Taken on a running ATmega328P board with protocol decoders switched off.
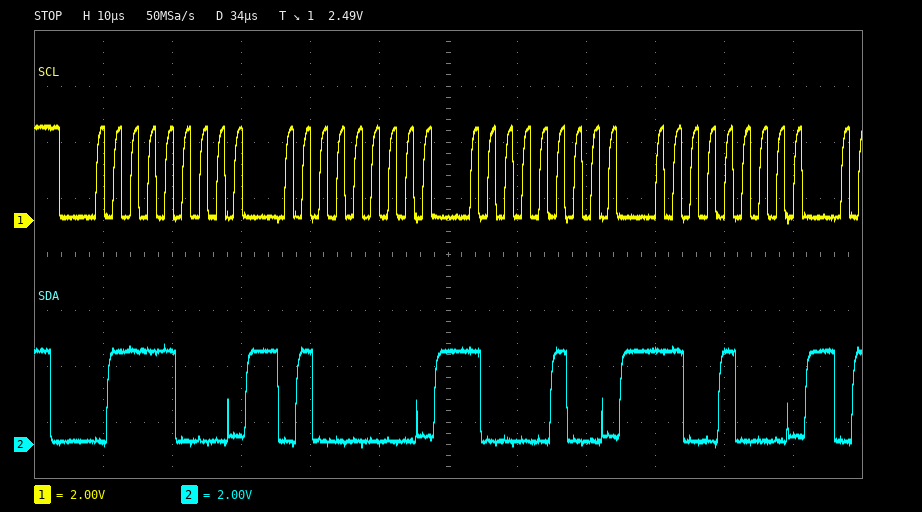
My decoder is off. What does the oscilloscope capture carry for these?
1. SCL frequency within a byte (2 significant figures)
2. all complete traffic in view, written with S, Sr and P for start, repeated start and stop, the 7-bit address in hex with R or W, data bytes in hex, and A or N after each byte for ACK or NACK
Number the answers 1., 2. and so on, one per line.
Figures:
1. 400 kHz
2. S 3CW A 40 A 84 A C8 A
